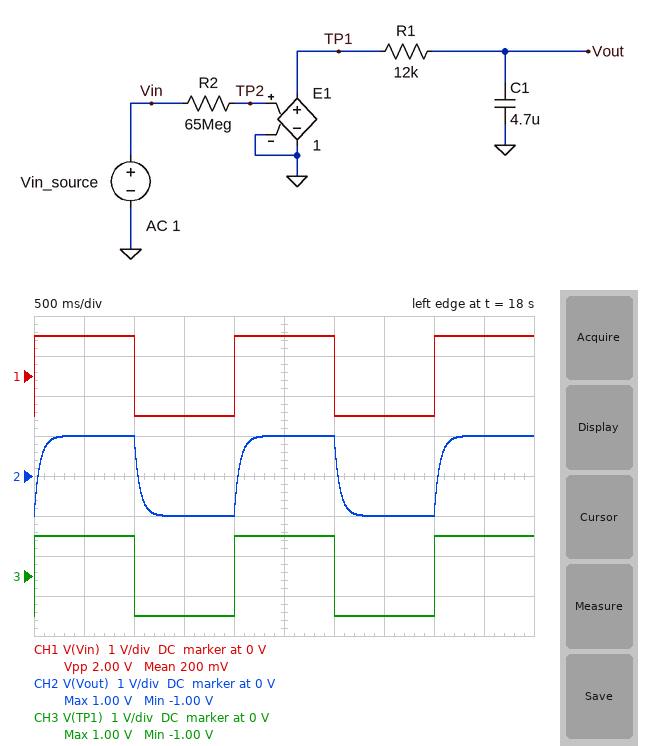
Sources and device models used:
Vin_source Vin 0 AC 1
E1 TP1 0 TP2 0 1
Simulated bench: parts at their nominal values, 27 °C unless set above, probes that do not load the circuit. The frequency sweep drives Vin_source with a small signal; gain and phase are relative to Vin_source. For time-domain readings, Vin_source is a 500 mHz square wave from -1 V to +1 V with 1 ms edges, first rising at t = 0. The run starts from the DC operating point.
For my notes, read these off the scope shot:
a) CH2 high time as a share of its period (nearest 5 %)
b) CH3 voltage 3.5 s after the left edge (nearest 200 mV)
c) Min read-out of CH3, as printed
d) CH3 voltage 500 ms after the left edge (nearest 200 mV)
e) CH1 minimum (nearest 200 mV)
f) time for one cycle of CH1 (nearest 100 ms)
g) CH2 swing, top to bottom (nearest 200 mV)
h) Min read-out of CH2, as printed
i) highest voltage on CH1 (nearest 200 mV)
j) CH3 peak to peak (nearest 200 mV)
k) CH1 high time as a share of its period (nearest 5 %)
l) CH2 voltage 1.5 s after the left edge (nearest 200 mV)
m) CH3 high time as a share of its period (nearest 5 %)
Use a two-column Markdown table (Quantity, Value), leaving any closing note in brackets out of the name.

| Quantity | Value |
|---|---|
| CH2 high time as a share of its period | 50 % |
| CH3 voltage 3.5 s after the left edge | -1.0 V |
| Min read-out of CH3, as printed | -1.00 V |
| CH3 voltage 500 ms after the left edge | 1.0 V |
| CH1 minimum | -1.0 V |
| time for one cycle of CH1 | 2.0 s |
| CH2 swing, top to bottom | 2.0 V |
| Min read-out of CH2, as printed | -1.00 V |
| highest voltage on CH1 | 1.0 V |
| CH3 peak to peak | 2.0 V |
| CH1 high time as a share of its period | 50 % |
| CH2 voltage 1.5 s after the left edge | -1.0 V |
| CH3 high time as a share of its period | 50 % |
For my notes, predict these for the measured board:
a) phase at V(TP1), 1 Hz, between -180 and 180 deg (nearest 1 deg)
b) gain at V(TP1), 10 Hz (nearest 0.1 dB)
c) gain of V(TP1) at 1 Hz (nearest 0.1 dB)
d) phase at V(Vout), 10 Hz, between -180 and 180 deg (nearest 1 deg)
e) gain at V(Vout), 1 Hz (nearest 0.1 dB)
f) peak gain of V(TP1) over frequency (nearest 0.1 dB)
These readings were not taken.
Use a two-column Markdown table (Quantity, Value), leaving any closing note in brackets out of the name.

| Quantity | Value |
|---|---|
| phase at V(TP1), 1 Hz, between -180 and 180 deg | 0 deg |
| gain at V(TP1), 10 Hz | 0 dB |
| gain of V(TP1) at 1 Hz | 0 dB |
| phase at V(Vout), 10 Hz, between -180 and 180 deg | -74 deg |
| gain at V(Vout), 1 Hz | -0.5 dB |
| peak gain of V(TP1) over frequency | 0 dB |
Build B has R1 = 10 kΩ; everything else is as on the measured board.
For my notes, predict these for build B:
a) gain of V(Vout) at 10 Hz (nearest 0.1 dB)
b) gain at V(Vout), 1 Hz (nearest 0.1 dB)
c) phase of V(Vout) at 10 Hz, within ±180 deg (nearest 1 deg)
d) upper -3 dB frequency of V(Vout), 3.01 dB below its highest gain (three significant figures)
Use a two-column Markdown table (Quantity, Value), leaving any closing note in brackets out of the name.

| Quantity | Value |
|---|---|
| gain of V(Vout) at 10 Hz | -9.9 dB |
| gain at V(Vout), 1 Hz | -0.4 dB |
| phase of V(Vout) at 10 Hz, within ±180 deg | -71 deg |
| upper -3 dB frequency of V(Vout), 3.01 dB below its highest gain | 3.39 Hz |
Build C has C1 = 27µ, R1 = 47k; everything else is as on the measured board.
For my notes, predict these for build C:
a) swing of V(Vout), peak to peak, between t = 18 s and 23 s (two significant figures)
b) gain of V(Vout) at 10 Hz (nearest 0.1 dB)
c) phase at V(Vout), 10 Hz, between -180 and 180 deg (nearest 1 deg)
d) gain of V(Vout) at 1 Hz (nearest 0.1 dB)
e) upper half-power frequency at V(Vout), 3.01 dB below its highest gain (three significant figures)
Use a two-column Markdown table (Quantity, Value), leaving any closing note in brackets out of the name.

| Quantity | Value |
|---|---|
| swing of V(Vout), peak to peak, between t = 18 s and 23 s | 750 mV |
| gain of V(Vout) at 10 Hz | -38.0 dB |
| phase at V(Vout), 10 Hz, between -180 and 180 deg | -89 deg |
| gain of V(Vout) at 1 Hz | -18.1 dB |
| upper half-power frequency at V(Vout), 3.01 dB below its highest gain | 125 mHz |
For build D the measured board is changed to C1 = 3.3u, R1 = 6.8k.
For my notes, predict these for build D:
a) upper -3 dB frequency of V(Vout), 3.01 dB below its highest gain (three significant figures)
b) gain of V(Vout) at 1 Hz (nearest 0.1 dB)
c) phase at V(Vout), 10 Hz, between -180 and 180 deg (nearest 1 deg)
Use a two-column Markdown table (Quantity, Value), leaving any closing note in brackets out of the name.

| Quantity | Value |
|---|---|
| upper -3 dB frequency of V(Vout), 3.01 dB below its highest gain | 7.09 Hz |
| gain of V(Vout) at 1 Hz | -0.1 dB |
| phase at V(Vout), 10 Hz, between -180 and 180 deg | -55 deg |
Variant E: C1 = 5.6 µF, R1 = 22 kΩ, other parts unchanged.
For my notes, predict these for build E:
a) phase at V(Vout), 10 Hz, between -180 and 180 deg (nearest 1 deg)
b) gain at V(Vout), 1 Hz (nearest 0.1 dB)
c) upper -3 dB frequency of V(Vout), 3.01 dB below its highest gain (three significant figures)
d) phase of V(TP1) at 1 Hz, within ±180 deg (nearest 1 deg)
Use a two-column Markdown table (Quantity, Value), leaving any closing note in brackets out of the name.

| Quantity | Value |
|---|---|
| phase at V(Vout), 10 Hz, between -180 and 180 deg | -83 deg |
| gain at V(Vout), 1 Hz | -2.0 dB |
| upper -3 dB frequency of V(Vout), 3.01 dB below its highest gain | 1.29 Hz |
| phase of V(TP1) at 1 Hz, within ±180 deg | 0 deg |
